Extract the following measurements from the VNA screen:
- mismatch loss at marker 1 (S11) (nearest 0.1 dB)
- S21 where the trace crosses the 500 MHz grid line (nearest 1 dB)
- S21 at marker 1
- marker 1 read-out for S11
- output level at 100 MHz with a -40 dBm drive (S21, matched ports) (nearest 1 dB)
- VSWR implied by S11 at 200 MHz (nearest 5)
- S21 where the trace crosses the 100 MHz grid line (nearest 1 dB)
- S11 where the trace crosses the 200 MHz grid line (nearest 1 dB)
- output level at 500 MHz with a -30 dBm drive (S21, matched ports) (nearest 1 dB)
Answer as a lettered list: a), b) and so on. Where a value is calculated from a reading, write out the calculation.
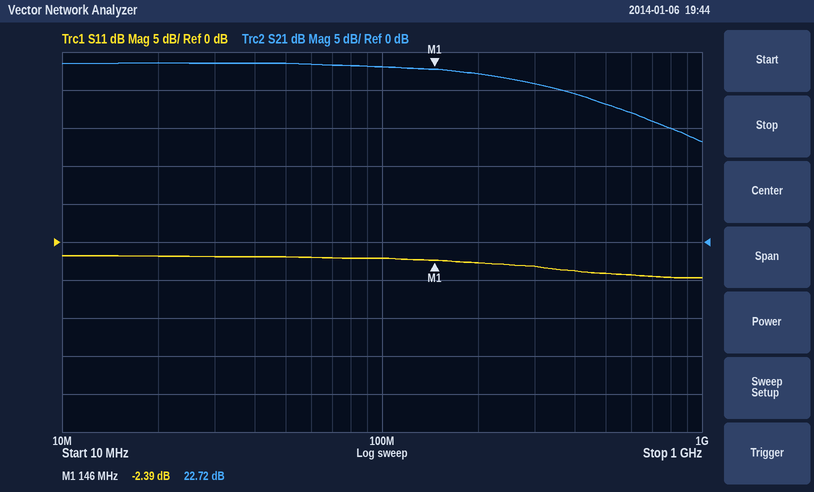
a) −10 log10(1 − 10^(-2.39/10)) ≈ 3.7 dB
b) 18 dB
c) 22.72 dB
d) -2.39 dB
e) -40 dBm + (23 dB) = -17 dBm
f) |Γ| = 10^(-3/20) = 0.7079; VSWR = (1 + 0.7079)/(1 − 0.7079) ≈ 5.85, so 5 to the nearest 5
g) 23 dB
h) -3 dB
i) -30 dBm + (18 dB) = -12 dBm
